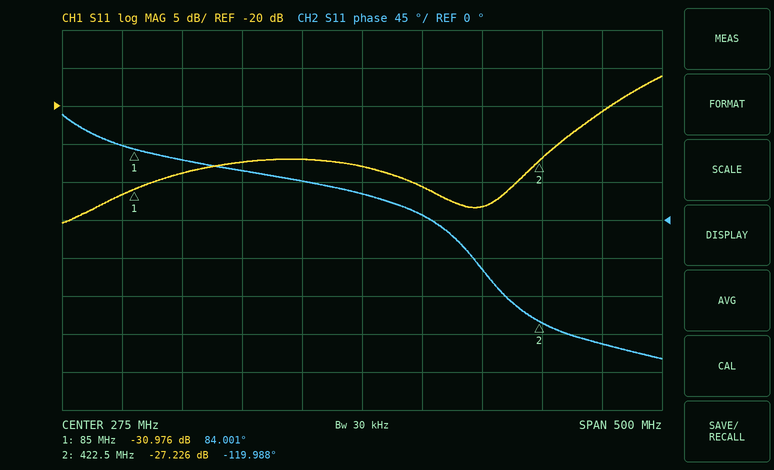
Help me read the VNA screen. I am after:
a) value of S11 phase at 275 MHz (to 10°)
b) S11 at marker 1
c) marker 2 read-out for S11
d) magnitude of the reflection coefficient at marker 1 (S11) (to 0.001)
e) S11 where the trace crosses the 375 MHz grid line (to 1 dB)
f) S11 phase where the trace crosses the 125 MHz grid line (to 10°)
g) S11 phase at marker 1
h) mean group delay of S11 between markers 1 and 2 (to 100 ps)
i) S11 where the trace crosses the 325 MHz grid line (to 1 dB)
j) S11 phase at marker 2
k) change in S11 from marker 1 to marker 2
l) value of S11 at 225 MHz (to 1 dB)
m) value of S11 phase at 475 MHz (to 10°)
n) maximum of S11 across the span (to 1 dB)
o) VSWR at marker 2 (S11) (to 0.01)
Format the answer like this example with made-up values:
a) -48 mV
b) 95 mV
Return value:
a) 30°
b) -30.976 dB
c) -27.226 dB
d) 0.028
e) -33 dB
f) 70°
g) 84.001°
h) 1.7 ns
i) -31 dB
j) -119.988°
k) 3.750 dB
l) -27 dB
m) -150°
n) -16 dB
o) 1.09
